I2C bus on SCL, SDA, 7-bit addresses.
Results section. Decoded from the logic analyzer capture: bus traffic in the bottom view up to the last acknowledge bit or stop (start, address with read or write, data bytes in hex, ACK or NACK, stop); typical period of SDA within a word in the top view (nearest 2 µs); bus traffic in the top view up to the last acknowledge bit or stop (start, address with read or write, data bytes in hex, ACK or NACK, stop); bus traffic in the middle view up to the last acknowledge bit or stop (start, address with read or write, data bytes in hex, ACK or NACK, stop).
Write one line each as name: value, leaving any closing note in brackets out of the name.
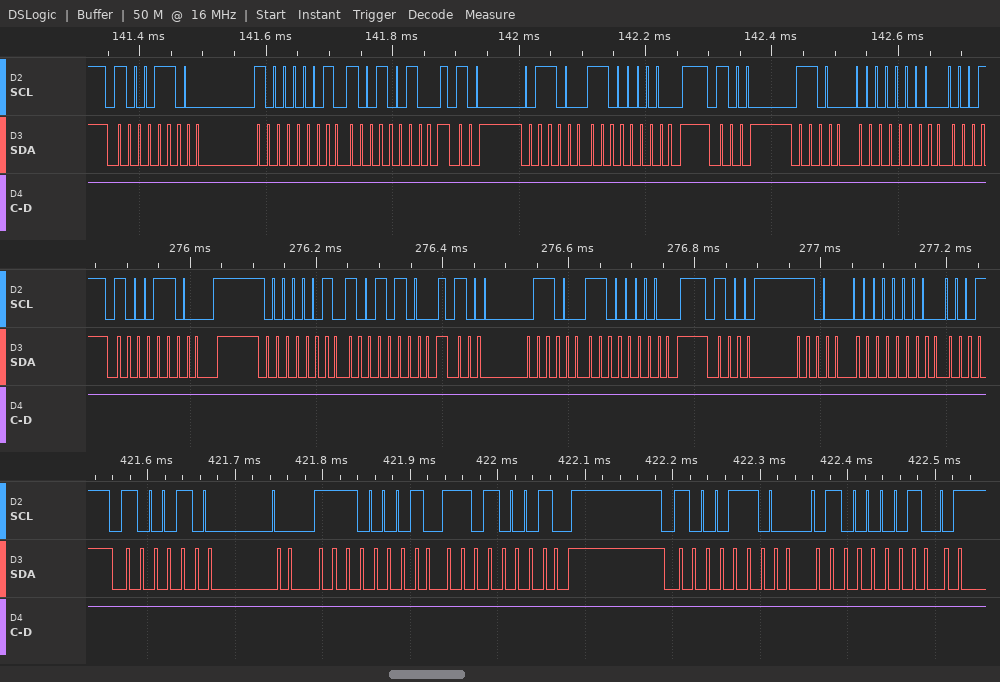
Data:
bus traffic in the bottom view up to the last acknowledge bit or stop: start, address 44 write ACK, E1 ACK, D1 ACK, stop, start, address 46 write ACK, 41 ACK
typical period of SDA within a word in the top view: 16 µs
bus traffic in the top view up to the last acknowledge bit or stop: start, address 46 write ACK, 81 ACK, 92 ACK, stop, start, address 46 write ACK, C0 ACK, stop, start, address 46 write ACK, 00 ACK
bus traffic in the middle view up to the last acknowledge bit or stop: start, address 46 write ACK, 81 ACK, 94 ACK, stop, start, address 46 write ACK, C0 ACK, stop, start, address 46 write ACK, 00 ACK
